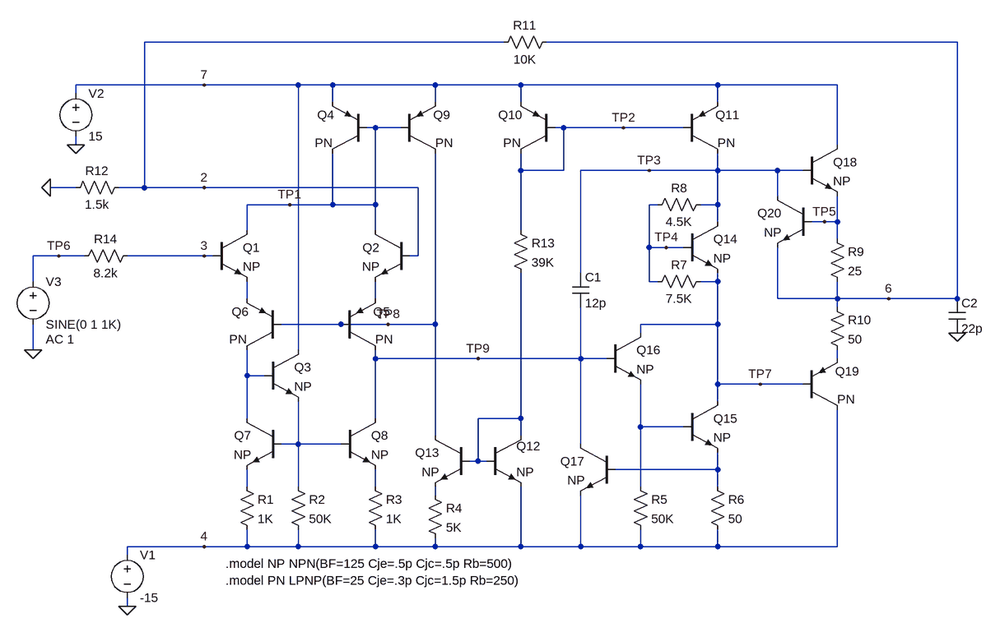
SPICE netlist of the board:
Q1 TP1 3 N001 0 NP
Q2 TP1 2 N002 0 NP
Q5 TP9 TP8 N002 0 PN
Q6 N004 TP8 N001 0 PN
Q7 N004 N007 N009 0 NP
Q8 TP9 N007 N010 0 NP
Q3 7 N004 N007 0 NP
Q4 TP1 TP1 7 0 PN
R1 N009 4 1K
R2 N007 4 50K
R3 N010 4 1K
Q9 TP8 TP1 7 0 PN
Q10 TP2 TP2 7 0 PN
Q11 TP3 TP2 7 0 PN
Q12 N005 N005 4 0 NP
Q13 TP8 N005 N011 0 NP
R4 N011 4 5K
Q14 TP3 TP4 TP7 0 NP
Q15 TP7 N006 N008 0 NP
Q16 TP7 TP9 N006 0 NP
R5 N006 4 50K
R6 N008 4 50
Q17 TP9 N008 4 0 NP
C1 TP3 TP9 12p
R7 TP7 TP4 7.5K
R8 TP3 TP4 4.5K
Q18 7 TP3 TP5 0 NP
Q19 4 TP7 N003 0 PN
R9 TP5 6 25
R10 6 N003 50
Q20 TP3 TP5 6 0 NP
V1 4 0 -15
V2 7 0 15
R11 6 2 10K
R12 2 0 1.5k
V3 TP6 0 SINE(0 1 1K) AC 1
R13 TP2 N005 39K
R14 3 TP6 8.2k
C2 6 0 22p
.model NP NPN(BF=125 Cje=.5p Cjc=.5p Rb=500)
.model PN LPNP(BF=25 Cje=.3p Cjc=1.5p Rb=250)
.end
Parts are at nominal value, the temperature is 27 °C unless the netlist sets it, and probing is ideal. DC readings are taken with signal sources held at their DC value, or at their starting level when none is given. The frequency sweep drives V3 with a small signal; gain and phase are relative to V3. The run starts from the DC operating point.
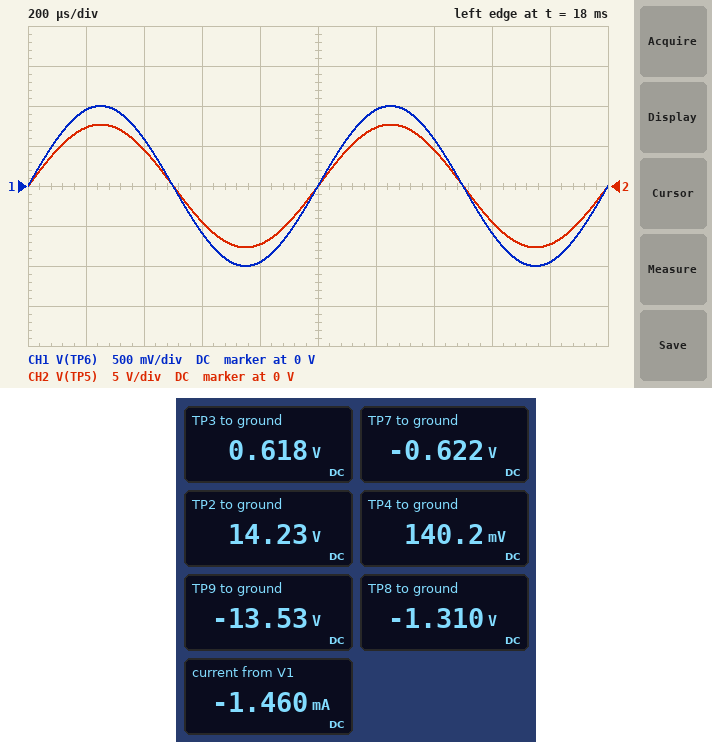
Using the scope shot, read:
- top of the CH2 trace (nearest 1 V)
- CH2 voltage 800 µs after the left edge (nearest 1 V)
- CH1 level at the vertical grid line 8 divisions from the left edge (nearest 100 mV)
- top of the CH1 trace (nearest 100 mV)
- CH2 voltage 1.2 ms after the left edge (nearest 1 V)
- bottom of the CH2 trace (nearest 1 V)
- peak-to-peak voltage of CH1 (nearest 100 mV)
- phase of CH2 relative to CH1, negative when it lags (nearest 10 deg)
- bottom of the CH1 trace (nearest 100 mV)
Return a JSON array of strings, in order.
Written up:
["8 V", "-7 V", "-600 mV", "1.0 V", "7 V", "-8 V", "2.0 V", "0 deg", "-1.0 V"]
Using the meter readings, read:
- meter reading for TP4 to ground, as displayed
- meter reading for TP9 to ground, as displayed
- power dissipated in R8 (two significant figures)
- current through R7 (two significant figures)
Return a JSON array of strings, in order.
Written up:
["140.2 mV", "-13.53 V", "51 µW", "100 µA"]
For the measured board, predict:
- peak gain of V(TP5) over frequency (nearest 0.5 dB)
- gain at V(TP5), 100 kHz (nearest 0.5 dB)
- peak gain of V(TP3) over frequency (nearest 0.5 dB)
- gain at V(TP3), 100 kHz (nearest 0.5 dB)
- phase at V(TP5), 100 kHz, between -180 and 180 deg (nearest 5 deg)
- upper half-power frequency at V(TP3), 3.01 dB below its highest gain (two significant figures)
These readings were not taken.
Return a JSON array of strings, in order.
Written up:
["17.5 dB", "17.0 dB", "21.0 dB", "20.0 dB", "-25 deg", "250 kHz"]
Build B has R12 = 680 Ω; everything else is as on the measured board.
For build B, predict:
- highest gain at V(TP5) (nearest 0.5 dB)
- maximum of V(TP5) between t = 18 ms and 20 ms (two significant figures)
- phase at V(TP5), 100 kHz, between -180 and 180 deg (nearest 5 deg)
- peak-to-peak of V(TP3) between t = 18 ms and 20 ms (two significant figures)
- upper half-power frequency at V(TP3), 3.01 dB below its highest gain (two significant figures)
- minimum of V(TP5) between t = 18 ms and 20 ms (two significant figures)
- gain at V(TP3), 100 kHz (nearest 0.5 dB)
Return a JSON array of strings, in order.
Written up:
["24.0 dB", "14 V", "-45 deg", "28 V", "110 kHz", "-13 V", "24.5 dB"]
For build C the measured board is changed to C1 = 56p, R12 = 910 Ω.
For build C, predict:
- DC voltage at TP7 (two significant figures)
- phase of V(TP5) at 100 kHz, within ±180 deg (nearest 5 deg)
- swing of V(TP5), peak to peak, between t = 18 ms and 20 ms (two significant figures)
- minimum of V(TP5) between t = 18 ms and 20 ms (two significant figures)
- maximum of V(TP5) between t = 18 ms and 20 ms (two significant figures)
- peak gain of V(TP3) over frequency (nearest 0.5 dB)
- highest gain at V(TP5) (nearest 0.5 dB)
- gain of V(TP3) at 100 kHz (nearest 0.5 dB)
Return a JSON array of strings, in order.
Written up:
["-620 mV", "-75 deg", "24 V", "-12 V", "12 V", "25.0 dB", "21.5 dB", "14.0 dB"]
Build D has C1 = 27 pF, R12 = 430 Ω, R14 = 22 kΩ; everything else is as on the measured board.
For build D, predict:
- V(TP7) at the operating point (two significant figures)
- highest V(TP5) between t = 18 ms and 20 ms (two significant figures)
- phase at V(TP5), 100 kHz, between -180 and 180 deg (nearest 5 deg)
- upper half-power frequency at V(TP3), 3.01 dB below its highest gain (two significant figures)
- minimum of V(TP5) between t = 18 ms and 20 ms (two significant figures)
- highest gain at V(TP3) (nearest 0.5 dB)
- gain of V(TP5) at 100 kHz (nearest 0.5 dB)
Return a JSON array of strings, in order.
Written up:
["-670 mV", "14 V", "-75 deg", "32 kHz", "-13 V", "30.5 dB", "17.5 dB"]
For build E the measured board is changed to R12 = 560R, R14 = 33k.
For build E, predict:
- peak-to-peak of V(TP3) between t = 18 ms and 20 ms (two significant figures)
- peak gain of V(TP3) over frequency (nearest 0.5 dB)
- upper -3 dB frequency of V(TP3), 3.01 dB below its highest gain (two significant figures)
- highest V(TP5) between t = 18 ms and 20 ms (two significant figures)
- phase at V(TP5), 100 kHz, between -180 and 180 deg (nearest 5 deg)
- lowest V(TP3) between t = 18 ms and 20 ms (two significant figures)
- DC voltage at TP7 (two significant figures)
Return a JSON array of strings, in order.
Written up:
["28 V", "28.5 dB", "95 kHz", "14 V", "-50 deg", "-13 V", "-680 mV"]
